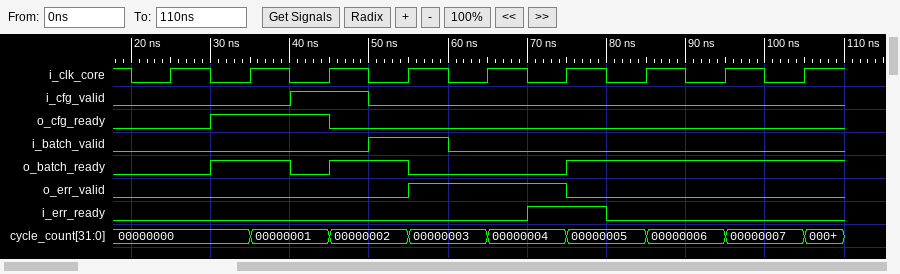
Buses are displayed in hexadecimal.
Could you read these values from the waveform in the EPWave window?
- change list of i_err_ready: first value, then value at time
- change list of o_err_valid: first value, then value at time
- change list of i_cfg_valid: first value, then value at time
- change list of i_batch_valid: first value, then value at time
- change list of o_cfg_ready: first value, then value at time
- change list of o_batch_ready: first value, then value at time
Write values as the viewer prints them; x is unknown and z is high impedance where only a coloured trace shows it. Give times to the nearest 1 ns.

0, 1 at 70 ns, 0 at 80 ns
0, 1 at 55 ns, 0 at 75 ns
0, 1 at 40 ns, 0 at 50 ns
0, 1 at 50 ns, 0 at 60 ns
0, 1 at 30 ns, 0 at 45 ns
0, 1 at 30 ns, 0 at 40 ns, 1 at 45 ns, 0 at 55 ns, 1 at 75 ns
